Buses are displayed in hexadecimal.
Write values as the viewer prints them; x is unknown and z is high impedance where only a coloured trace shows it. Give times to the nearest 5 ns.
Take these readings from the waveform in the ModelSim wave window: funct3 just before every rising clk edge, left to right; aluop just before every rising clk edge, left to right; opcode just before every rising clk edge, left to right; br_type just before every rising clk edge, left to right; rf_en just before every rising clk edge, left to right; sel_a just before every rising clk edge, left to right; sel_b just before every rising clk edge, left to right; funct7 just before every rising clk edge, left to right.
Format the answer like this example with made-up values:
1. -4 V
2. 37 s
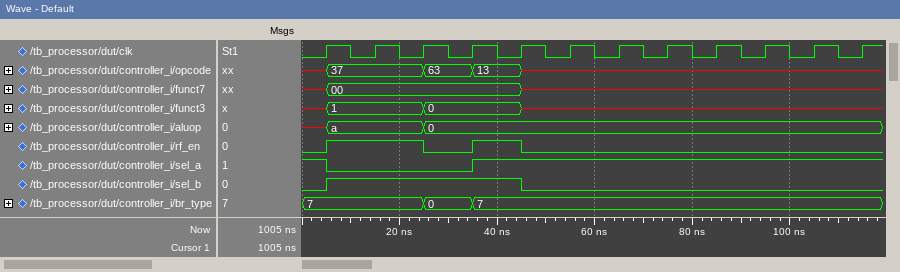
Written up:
1. x, 1, 1, 0, 0, x, x, x, x, x, x, x
2. x, a, a, 0, 0, 0, 0, 0, 0, 0, 0, 0
3. x, 37, 37, 63, 13, x, x, x, x, x, x, x
4. 7, 7, 7, 0, 7, 7, 7, 7, 7, 7, 7, 7
5. 0 1 1 0 1 0 0 0 0 0 0 0
6. 1 0 0 0 1 1 1 1 1 1 1 1
7. 0 1 1 1 1 0 0 0 0 0 0 0
8. x, 00, 00, 00, 00, x, x, x, x, x, x, x
